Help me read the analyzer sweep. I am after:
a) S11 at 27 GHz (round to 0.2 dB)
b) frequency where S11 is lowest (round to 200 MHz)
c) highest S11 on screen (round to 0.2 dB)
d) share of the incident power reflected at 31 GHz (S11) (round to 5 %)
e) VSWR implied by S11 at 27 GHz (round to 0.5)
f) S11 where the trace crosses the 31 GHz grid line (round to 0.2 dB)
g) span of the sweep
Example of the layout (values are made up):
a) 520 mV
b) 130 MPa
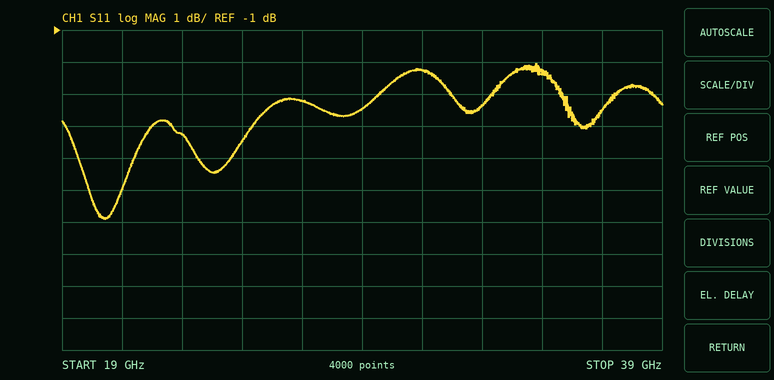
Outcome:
a) -3.2 dB
b) 20.4 GHz
c) -2.0 dB
d) 60 %
e) 5.5
f) -2.2 dB
g) 20 GHz
